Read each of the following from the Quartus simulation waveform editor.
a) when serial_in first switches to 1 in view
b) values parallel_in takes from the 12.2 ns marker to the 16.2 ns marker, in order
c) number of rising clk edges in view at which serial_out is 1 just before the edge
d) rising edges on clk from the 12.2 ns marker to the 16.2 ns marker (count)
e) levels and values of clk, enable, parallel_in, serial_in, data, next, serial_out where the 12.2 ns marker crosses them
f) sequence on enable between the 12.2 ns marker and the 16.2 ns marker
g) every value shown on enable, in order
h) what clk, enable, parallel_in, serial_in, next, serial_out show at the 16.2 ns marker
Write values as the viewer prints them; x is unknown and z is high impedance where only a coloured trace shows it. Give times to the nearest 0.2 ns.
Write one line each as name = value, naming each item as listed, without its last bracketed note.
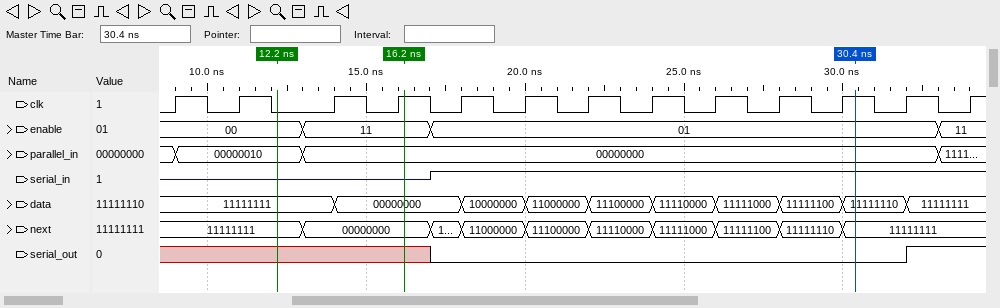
when serial_in first switches to 1 in view = 17 ns
values parallel_in takes from the 12.2 ns marker to the 16.2 ns marker, in order = 00000010, 00000000
number of rising clk edges in view at which serial_out is 1 just before the edge = 1
rising edges on clk from the 12.2 ns marker to the 16.2 ns marker = 2
levels and values of clk, enable, parallel_in, serial_in, data, next, serial_out where the 12.2 ns marker crosses them = clk=0, enable=00, parallel_in=00000010, serial_in=z, data=11111111, next=11111111, serial_out=x
sequence on enable between the 12.2 ns marker and the 16.2 ns marker = 00, 11
every value shown on enable, in order = 00, 11, 01, 11
what clk, enable, parallel_in, serial_in, next, serial_out show at the 16.2 ns marker = clk=1, enable=11, parallel_in=00000000, serial_in=z, next=00000000, serial_out=x
